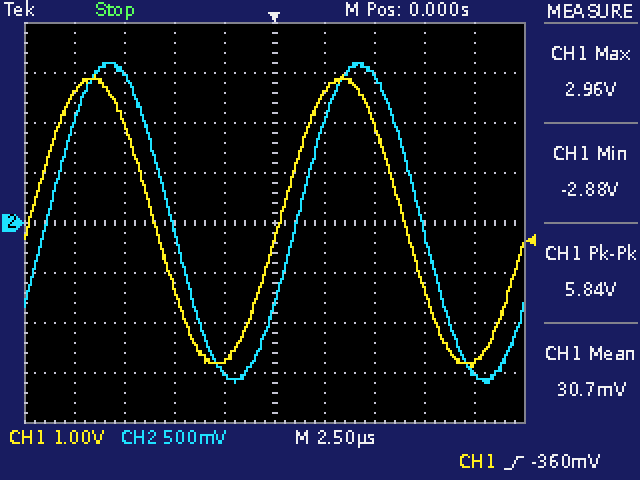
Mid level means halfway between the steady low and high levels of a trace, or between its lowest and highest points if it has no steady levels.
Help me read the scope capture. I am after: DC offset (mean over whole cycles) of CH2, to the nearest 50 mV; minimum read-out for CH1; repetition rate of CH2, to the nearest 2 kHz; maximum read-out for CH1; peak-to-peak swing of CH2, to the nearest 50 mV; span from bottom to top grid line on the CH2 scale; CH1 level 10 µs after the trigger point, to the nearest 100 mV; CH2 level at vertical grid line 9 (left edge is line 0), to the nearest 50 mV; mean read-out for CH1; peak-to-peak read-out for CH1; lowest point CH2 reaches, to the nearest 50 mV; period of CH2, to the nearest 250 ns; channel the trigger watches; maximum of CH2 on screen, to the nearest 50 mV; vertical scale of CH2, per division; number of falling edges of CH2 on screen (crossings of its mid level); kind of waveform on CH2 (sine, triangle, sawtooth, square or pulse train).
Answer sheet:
0 mV
-2.88 V
80 kHz
2.96 V
3.20 V
4 V
-2.8 V
-1.50 V
30.7 mV
5.84 V
-1.60 V
12.50 µs
CH1
1.60 V
500 mV
2
sine
